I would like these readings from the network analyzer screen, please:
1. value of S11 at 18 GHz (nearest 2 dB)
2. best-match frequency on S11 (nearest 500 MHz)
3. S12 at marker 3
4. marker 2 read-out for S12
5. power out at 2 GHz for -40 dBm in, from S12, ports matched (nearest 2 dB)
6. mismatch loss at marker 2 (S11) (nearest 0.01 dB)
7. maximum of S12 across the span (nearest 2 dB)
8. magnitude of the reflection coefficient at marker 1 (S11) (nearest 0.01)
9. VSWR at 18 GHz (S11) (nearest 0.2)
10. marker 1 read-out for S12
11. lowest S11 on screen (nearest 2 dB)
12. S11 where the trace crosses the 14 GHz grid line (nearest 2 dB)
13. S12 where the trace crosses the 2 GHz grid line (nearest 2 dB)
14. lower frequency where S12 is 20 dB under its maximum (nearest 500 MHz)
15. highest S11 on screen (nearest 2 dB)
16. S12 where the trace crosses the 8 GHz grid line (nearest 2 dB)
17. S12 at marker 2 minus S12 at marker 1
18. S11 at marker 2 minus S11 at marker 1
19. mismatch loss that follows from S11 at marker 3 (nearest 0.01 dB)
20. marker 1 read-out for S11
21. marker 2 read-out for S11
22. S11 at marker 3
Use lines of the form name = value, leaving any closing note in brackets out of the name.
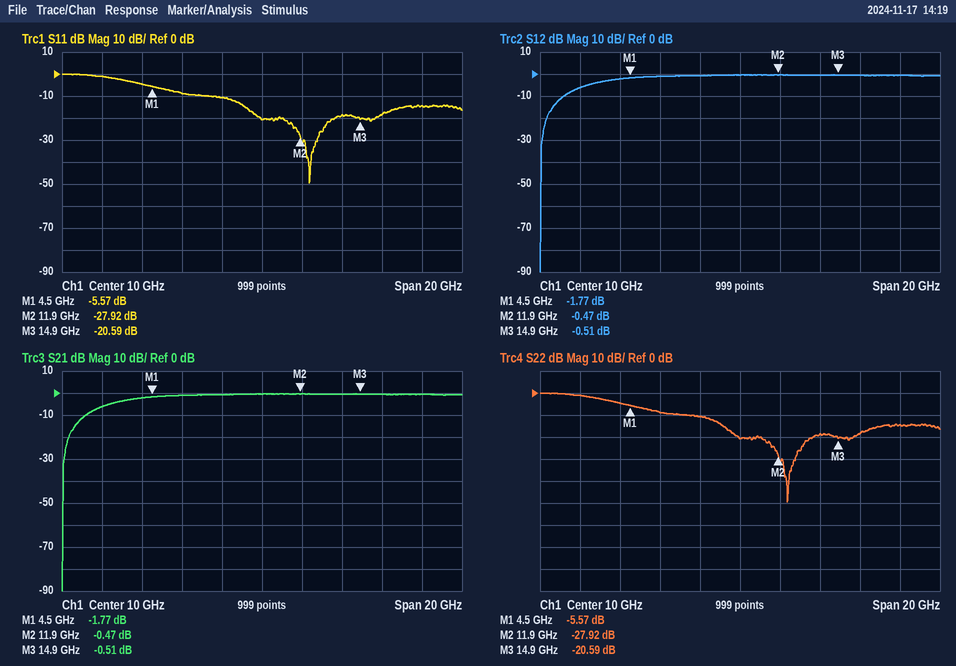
value of S11 at 18 GHz = -14 dB
best-match frequency on S11 = 12.5 GHz
S12 at marker 3 = -0.51 dB
marker 2 read-out for S12 = -0.47 dB
power out at 2 GHz for -40 dBm in, from S12, ports matched = -46 dBm
mismatch loss at marker 2 (S11) = 0.01 dB
maximum of S12 across the span = 0 dB
magnitude of the reflection coefficient at marker 1 (S11) = 0.53
VSWR at 18 GHz (S11) = 1.4
marker 1 read-out for S12 = -1.77 dB
lowest S11 on screen = -50 dB
S11 where the trace crosses the 14 GHz grid line = -18 dB
S12 where the trace crosses the 2 GHz grid line = -6 dB
lower frequency where S12 is 20 dB under its maximum = 500 MHz
highest S11 on screen = 0 dB
S12 where the trace crosses the 8 GHz grid line = 0 dB
S12 at marker 2 minus S12 at marker 1 = 1.30 dB
S11 at marker 2 minus S11 at marker 1 = -22.35 dB
mismatch loss that follows from S11 at marker 3 = 0.04 dB
marker 1 read-out for S11 = -5.57 dB
marker 2 read-out for S11 = -27.92 dB
S11 at marker 3 = -20.59 dB
